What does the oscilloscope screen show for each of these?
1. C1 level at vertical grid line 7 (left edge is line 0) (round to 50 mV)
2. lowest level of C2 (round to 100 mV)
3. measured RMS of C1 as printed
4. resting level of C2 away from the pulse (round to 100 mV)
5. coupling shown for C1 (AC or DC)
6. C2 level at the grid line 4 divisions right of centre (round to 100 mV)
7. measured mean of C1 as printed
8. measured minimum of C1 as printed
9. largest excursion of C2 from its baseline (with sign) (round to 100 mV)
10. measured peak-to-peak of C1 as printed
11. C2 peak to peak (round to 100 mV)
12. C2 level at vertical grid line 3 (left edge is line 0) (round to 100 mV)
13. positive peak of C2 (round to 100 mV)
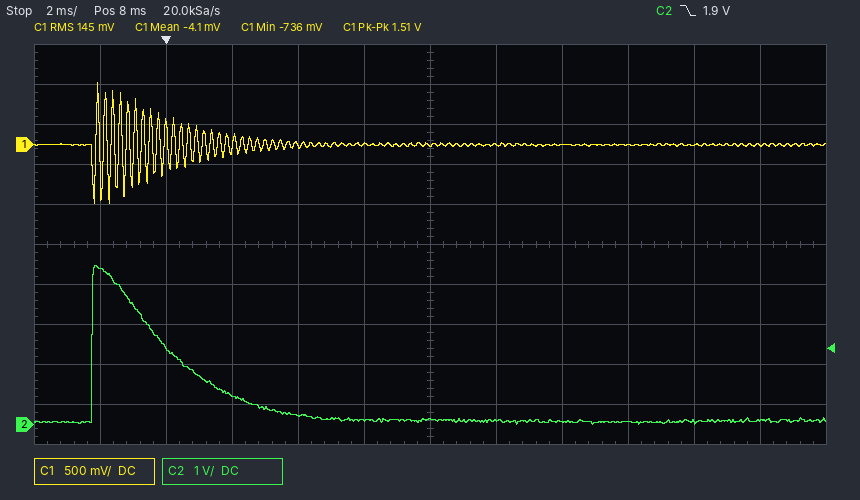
0 mV
0.0 V
145 mV
100 mV
DC
100 mV
-4.1 mV
-736 mV
+3.9 V
1.51 V
4.0 V
700 mV
4.0 V
